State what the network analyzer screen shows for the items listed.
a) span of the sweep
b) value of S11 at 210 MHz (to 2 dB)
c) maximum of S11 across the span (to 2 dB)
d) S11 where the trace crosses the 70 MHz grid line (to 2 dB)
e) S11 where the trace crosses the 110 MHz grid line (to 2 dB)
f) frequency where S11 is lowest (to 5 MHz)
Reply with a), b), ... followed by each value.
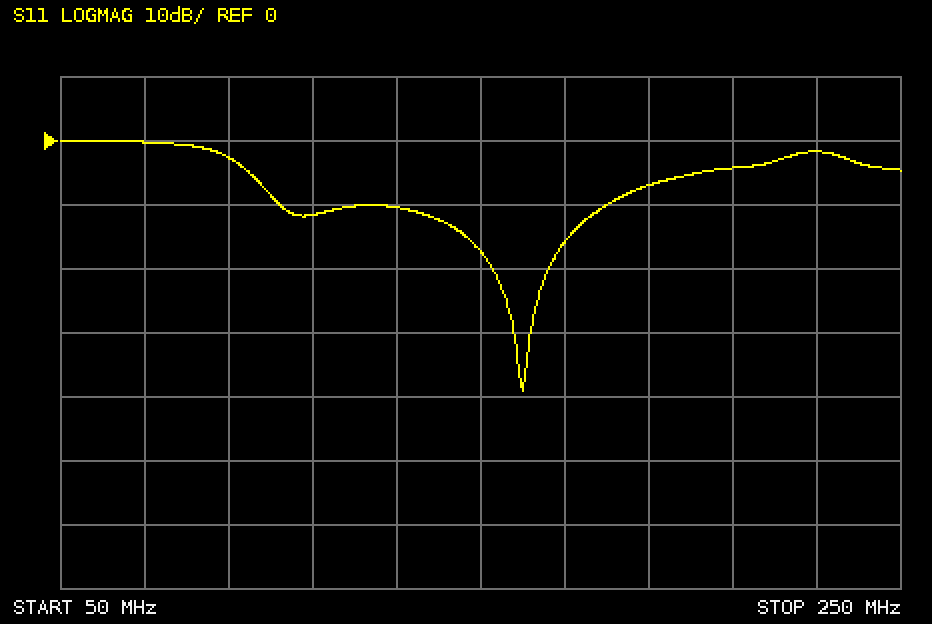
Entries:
a) 200 MHz
b) -4 dB
c) 0 dB
d) 0 dB
e) -12 dB
f) 160 MHz
